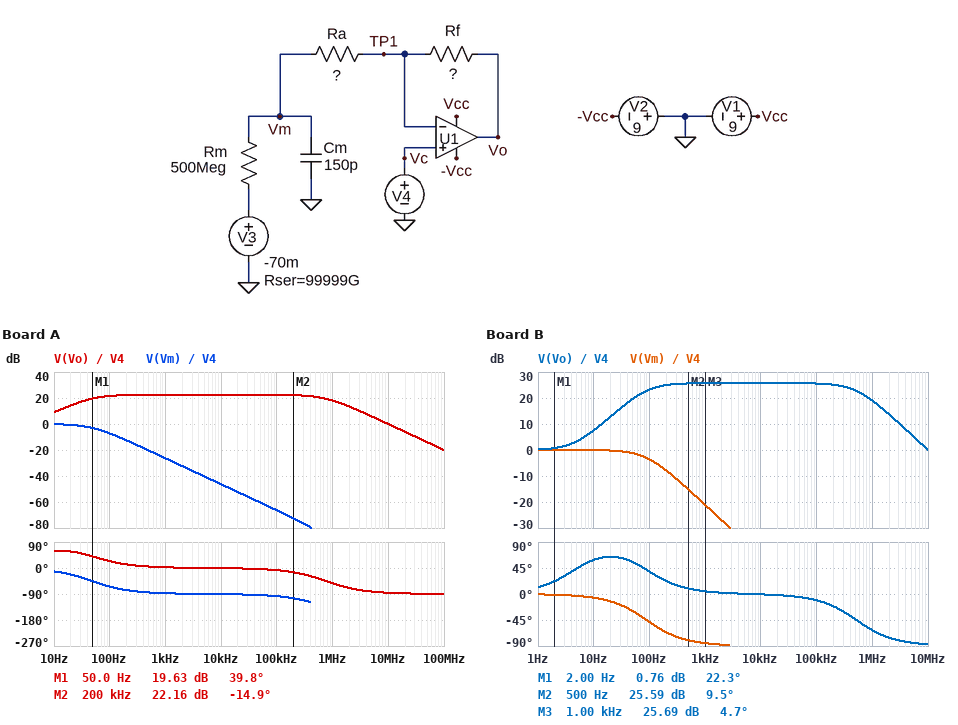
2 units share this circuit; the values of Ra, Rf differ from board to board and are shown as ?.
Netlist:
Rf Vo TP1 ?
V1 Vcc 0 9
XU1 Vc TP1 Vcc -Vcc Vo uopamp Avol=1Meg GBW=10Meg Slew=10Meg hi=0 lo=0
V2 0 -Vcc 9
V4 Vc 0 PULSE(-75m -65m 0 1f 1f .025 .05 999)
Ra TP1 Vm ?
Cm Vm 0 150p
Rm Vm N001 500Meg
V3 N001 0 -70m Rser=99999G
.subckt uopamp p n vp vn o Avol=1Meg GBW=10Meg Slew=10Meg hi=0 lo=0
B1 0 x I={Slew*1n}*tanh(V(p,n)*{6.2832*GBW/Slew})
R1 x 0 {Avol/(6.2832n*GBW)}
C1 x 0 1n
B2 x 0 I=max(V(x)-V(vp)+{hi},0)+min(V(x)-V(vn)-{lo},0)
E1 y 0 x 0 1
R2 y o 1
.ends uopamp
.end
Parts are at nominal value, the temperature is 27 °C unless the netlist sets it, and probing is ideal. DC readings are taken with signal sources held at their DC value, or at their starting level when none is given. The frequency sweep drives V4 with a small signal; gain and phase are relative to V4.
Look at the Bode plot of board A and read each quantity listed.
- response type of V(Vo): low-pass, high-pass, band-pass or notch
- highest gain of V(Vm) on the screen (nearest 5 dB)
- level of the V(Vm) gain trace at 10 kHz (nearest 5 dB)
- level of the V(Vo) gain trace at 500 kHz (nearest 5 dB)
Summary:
band-pass
0 dB
-45 dB
20 dB
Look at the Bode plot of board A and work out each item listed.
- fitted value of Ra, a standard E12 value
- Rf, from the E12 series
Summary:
22 MΩ
270 MΩ
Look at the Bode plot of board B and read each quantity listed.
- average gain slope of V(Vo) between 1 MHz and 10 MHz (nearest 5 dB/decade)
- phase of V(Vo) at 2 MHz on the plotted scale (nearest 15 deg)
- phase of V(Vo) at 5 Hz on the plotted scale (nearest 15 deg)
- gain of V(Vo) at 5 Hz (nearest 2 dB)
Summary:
-20 dB/decade
-75 deg
45 deg
4 dB
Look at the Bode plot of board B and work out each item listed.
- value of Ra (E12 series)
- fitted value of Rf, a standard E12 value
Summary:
12 MΩ
220 MΩ
